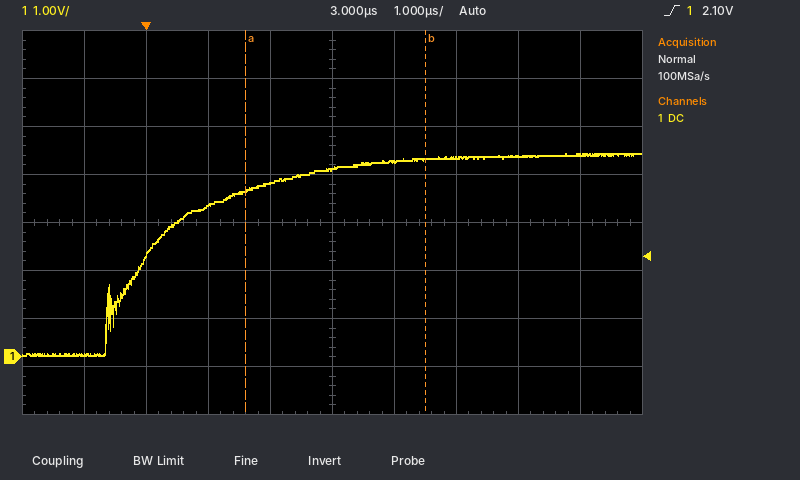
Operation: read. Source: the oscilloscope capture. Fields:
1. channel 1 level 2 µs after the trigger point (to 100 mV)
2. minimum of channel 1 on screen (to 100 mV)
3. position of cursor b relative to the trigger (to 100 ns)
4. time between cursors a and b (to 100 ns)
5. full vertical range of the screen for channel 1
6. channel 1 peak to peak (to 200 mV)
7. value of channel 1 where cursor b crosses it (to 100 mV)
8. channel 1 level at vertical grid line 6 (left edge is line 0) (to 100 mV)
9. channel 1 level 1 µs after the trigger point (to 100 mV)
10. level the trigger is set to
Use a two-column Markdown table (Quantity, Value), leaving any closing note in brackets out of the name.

| Quantity | Value |
|---|---|
| channel 1 level 2 µs after the trigger point | 3.6 V |
| minimum of channel 1 on screen | 0.0 V |
| position of cursor b relative to the trigger | +4.5 µs |
| time between cursors a and b | 2.9 µs |
| full vertical range of the screen for channel 1 | 8 V |
| channel 1 peak to peak | 4.2 V |
| value of channel 1 where cursor b crosses it | 4.1 V |
| channel 1 level at vertical grid line 6 (left edge is line 0) | 4.1 V |
| channel 1 level 1 µs after the trigger point | 3.2 V |
| level the trigger is set to | 2.10 V |
